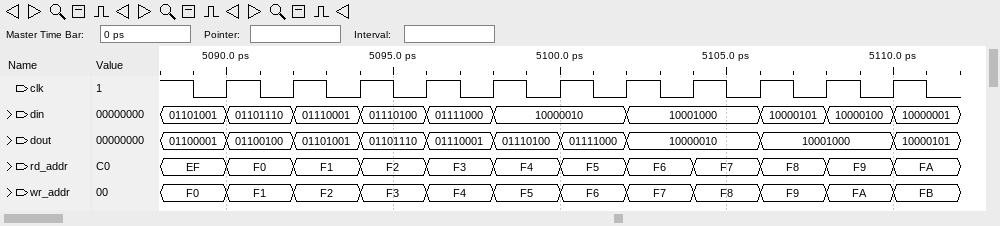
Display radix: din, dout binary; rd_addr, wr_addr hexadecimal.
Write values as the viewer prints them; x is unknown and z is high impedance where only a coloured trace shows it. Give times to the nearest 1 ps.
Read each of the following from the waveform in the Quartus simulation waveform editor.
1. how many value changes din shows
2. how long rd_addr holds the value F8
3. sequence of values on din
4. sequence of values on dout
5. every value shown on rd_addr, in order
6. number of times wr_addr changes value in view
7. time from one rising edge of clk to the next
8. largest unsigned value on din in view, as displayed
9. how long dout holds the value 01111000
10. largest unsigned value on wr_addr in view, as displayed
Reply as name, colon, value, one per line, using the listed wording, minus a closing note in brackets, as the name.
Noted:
how many value changes din shows: 9
how long rd_addr holds the value F8: 2 ps
sequence of values on din: 01101001, 01101110, 01110001, 01110100, 01111000, 10000010, 10001000, 10000101, 10000100, 10000001
sequence of values on dout: 01100001, 01100100, 01101001, 01101110, 01110001, 01110100, 01111000, 10000010, 10001000, 10000101
every value shown on rd_addr, in order: EF, F0, F1, F2, F3, F4, F5, F6, F7, F8, F9, FA
number of times wr_addr changes value in view: 11
time from one rising edge of clk to the next: 2 ps
largest unsigned value on din in view, as displayed: 10001000
how long dout holds the value 01111000: 2 ps
largest unsigned value on wr_addr in view, as displayed: FB
